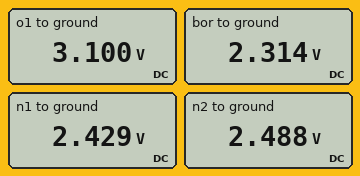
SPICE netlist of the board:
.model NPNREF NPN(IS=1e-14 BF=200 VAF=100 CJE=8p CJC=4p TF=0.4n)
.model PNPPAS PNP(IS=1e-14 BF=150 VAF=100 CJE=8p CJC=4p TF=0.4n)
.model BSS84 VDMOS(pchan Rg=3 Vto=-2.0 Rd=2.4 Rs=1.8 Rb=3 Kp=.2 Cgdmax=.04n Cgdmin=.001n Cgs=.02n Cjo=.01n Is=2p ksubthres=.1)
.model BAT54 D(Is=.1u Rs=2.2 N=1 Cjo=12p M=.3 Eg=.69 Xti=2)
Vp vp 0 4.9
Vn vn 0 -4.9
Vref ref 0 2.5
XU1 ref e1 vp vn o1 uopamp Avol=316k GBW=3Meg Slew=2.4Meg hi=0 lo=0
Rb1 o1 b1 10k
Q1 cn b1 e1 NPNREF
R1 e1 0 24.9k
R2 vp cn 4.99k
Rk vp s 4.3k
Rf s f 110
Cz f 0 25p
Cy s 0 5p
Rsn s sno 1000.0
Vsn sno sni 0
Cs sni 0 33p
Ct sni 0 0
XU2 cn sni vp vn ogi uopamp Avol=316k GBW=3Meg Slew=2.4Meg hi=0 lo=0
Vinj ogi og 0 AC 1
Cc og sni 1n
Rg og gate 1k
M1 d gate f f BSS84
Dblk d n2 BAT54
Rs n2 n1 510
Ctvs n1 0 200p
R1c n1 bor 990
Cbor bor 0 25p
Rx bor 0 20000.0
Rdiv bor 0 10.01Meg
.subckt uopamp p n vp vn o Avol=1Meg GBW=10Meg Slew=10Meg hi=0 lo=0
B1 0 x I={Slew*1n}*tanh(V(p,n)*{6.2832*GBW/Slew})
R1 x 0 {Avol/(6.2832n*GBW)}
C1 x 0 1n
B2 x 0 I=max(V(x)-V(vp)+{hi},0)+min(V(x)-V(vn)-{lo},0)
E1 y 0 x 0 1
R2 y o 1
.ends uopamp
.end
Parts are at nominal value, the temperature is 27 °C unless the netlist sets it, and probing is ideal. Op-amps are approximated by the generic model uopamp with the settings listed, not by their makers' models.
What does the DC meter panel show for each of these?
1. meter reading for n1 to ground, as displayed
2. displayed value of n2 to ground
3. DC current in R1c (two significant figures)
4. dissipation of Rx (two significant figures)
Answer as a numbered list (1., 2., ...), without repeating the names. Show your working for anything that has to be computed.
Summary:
1. 2.429 V
2. 2.488 V
3. (2.429 V - 2.314 V) / 990 Ω = 120 µA
4. (2.314 V)^2 / 20 kΩ = 270 µW
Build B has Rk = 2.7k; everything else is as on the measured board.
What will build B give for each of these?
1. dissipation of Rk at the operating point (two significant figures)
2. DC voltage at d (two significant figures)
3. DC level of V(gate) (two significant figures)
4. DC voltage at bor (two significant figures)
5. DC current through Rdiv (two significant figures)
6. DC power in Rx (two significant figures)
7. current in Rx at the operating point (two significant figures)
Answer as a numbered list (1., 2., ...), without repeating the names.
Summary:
1. 92 µW
2. 4.2 V
3. 2.4 V
4. 3.7 V
5. 370 nA
6. 680 µW
7. 180 µA
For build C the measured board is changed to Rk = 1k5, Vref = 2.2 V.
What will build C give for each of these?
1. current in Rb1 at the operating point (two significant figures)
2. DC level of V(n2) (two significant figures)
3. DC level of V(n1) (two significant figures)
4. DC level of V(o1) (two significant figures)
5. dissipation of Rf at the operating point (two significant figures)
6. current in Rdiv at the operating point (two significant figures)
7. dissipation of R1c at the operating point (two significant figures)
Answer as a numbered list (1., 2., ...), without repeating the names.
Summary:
1. 430 nA
2. 4.4 V
3. 4.3 V
4. 2.8 V
5. 4.6 µW
6. 410 nA
7. 41 µW
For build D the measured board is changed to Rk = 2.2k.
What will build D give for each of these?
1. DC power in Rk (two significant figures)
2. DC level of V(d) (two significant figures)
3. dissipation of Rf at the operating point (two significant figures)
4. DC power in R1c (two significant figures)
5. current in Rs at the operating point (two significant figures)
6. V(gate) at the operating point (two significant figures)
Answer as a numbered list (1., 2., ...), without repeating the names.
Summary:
1. 86 µW
2. 4.4 V
3. 4.3 µW
4. 39 µW
5. 200 µA
6. -4.9 V
